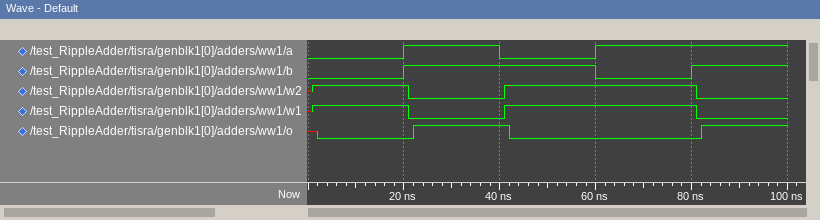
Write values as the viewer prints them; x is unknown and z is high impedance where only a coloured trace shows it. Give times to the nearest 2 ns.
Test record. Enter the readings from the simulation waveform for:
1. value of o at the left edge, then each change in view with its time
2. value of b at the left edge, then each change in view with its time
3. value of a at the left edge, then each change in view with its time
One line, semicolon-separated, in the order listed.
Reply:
x, 0 at 2 ns, 1 at 22 ns, 0 at 42 ns, 1 at 82 ns; 0, 1 at 20 ns, 0 at 60 ns, 1 at 80 ns; 0, 1 at 20 ns, 0 at 40 ns, 1 at 60 ns
